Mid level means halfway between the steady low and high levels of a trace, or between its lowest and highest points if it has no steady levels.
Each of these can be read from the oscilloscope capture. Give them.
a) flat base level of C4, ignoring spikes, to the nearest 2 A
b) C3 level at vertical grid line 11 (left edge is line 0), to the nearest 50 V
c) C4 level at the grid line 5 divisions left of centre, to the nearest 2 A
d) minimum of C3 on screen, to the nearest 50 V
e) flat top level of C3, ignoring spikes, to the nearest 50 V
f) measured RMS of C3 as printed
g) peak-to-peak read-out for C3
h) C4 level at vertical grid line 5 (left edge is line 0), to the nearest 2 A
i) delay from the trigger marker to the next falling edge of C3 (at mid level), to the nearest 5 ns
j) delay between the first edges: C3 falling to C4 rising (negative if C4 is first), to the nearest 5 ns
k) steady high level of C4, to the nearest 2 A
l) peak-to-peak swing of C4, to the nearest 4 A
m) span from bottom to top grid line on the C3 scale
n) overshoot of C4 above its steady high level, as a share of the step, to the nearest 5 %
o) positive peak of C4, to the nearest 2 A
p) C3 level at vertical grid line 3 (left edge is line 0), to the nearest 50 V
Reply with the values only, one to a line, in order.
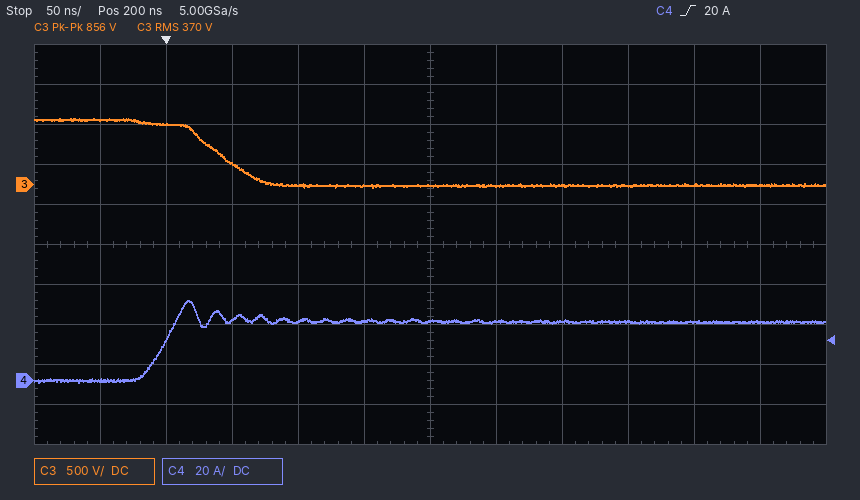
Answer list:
0 A
0 V
0 A
-50 V
800 V
370 V
856 V
30 A
40 ns
-45 ns
30 A
40 A
5 kV
35 %
40 A
250 V
